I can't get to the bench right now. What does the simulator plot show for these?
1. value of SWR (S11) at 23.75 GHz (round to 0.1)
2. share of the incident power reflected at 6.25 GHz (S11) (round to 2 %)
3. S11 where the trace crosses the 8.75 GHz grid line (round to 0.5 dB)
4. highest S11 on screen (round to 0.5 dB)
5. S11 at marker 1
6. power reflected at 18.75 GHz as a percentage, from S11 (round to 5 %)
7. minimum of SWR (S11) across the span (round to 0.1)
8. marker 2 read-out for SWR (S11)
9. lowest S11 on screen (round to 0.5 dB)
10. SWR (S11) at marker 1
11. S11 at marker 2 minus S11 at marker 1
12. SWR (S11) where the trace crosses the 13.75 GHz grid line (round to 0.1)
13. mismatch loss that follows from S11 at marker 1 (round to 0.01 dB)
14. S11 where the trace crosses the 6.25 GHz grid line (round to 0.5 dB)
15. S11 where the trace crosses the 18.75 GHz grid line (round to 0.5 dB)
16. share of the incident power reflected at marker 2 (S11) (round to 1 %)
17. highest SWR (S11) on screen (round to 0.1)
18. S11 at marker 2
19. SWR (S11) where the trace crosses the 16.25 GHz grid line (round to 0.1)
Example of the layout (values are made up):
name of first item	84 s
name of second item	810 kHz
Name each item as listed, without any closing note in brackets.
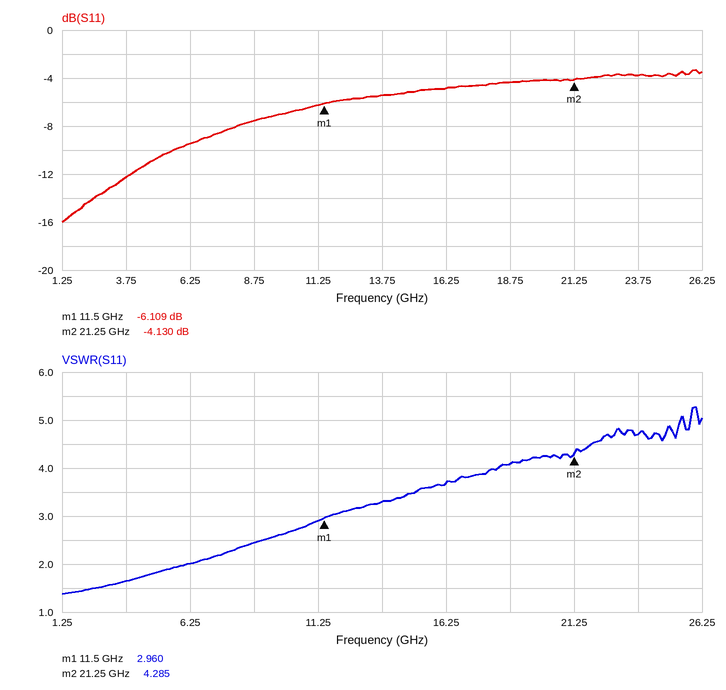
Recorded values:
value of SWR (S11) at 23.75 GHz	4.7
share of the incident power reflected at 6.25 GHz (S11)	12 %
S11 where the trace crosses the 8.75 GHz grid line	-7.5 dB
highest S11 on screen	-3.5 dB
S11 at marker 1	-6.109 dB
power reflected at 18.75 GHz as a percentage, from S11	35 %
minimum of SWR (S11) across the span	1.4
marker 2 read-out for SWR	4.285
lowest S11 on screen	-16.0 dB
SWR (S11) at marker 1	2.960
S11 at marker 2 minus S11 at marker 1	1.979 dB
SWR (S11) where the trace crosses the 13.75 GHz grid line	3.3
mismatch loss that follows from S11 at marker 1	1.22 dB
S11 where the trace crosses the 6.25 GHz grid line	-9.5 dB
S11 where the trace crosses the 18.75 GHz grid line	-4.5 dB
share of the incident power reflected at marker 2 (S11)	39 %
highest SWR (S11) on screen	5.3
S11 at marker 2	-4.130 dB
SWR (S11) where the trace crosses the 16.25 GHz grid line	3.7
